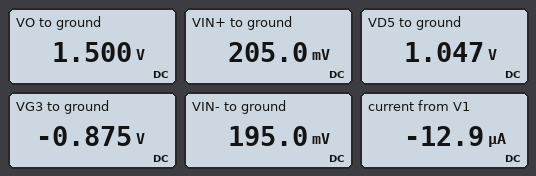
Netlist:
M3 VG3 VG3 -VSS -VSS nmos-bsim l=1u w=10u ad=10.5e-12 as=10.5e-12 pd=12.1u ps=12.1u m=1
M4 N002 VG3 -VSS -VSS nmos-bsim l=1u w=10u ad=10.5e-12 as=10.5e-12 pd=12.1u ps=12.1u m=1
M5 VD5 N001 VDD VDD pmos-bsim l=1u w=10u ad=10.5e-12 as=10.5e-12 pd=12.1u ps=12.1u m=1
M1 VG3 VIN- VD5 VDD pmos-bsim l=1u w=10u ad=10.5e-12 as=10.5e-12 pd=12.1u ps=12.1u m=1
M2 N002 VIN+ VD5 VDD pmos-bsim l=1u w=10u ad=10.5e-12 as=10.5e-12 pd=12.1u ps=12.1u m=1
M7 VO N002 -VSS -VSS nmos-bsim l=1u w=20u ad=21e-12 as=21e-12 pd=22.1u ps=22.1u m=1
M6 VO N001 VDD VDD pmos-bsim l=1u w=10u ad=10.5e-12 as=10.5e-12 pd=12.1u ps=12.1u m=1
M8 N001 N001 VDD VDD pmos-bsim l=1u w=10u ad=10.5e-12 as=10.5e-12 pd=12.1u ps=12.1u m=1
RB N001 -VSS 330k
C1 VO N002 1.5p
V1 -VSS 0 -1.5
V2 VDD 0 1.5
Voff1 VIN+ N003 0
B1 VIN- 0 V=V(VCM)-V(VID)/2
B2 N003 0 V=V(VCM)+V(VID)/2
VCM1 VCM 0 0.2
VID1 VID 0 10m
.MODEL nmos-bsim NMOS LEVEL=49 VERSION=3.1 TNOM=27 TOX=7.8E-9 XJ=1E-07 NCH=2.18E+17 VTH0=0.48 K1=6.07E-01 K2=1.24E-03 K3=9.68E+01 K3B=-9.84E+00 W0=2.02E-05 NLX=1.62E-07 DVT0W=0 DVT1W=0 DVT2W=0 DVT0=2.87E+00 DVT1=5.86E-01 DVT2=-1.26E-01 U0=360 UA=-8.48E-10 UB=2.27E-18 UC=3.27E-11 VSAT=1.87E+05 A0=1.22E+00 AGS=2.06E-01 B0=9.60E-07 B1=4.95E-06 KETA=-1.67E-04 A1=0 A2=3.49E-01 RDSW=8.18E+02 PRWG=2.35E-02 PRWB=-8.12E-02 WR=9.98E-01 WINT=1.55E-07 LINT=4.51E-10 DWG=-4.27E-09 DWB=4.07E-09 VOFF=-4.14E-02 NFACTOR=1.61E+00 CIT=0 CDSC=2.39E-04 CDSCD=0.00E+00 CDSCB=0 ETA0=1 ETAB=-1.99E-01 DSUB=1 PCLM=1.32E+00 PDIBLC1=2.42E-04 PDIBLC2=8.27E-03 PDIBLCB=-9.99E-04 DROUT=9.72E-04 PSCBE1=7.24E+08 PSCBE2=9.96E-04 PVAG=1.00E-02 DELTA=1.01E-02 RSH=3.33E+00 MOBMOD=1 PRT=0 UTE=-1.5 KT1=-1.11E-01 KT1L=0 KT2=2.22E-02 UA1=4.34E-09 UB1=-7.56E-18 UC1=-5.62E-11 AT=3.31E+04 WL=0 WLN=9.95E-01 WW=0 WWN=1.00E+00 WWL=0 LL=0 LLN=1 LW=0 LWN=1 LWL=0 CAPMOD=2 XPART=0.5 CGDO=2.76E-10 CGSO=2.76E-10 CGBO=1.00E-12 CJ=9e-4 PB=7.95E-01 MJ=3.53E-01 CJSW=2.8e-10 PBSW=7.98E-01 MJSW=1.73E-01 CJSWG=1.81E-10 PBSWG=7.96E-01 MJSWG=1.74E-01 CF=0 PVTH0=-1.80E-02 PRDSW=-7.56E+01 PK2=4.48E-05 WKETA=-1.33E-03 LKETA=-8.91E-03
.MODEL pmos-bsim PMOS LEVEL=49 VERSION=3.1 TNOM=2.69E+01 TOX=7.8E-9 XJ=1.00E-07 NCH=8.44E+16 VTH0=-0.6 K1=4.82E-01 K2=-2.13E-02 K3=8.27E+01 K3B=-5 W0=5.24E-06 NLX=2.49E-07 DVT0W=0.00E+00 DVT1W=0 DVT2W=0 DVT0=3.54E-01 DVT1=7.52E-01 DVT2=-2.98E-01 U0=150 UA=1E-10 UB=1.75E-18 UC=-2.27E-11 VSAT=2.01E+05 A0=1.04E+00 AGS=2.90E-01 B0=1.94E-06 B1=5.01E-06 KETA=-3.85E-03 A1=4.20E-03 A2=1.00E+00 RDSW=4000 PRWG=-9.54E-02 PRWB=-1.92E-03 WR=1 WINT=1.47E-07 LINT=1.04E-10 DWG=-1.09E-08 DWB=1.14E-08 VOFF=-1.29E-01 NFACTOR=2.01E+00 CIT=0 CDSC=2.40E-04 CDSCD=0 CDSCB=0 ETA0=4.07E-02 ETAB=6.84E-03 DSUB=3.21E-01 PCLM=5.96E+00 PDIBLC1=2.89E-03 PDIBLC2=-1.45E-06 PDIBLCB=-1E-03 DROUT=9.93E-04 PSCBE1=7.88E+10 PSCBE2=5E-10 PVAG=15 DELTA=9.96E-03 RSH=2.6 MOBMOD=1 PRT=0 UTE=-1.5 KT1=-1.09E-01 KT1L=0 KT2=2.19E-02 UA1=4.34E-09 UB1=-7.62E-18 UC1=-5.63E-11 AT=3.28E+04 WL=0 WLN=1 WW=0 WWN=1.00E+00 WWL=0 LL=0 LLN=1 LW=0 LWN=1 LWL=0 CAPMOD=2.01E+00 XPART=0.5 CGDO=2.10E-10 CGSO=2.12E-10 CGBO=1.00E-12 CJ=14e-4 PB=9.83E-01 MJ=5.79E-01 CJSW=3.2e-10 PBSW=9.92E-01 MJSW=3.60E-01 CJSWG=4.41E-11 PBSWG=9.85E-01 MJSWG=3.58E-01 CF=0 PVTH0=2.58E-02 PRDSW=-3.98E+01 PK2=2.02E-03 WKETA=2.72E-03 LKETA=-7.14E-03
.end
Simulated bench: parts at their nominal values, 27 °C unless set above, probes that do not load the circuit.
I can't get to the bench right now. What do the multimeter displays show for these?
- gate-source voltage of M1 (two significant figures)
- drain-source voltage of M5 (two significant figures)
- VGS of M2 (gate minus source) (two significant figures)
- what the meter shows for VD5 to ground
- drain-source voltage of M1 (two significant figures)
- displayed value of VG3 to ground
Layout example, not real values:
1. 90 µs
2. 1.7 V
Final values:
1. -850 mV
2. -450 mV
3. -840 mV
4. 1.047 V
5. -1.9 V
6. -0.875 V
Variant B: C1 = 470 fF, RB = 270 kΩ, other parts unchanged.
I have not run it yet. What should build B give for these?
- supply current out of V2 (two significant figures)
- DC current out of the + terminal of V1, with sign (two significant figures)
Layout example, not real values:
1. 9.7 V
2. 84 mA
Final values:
1. 16 µA
2. -16 µA
